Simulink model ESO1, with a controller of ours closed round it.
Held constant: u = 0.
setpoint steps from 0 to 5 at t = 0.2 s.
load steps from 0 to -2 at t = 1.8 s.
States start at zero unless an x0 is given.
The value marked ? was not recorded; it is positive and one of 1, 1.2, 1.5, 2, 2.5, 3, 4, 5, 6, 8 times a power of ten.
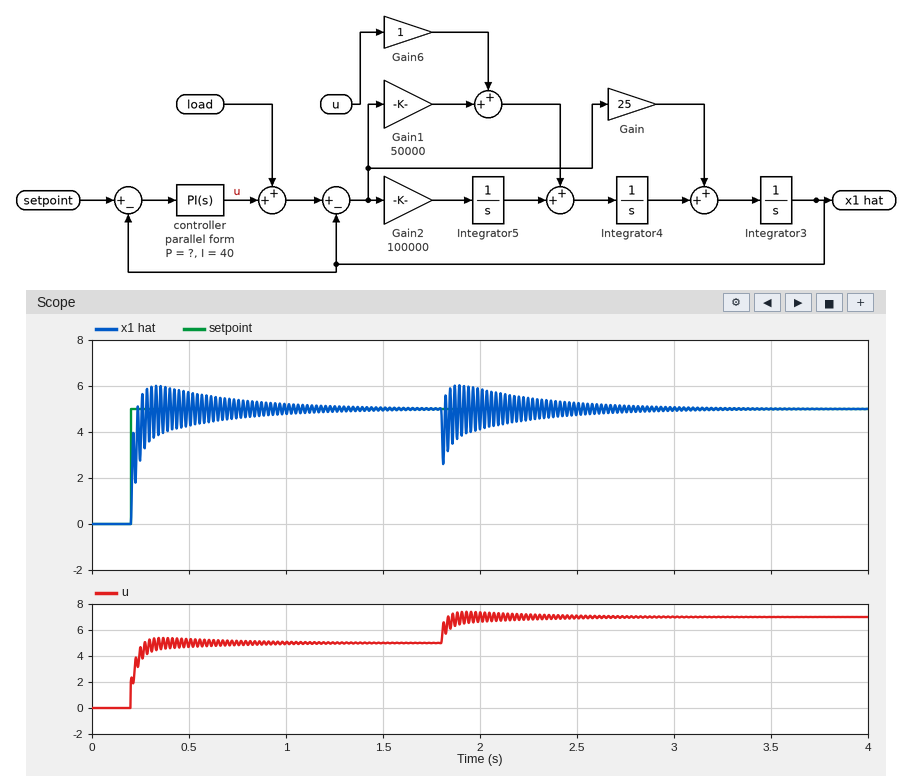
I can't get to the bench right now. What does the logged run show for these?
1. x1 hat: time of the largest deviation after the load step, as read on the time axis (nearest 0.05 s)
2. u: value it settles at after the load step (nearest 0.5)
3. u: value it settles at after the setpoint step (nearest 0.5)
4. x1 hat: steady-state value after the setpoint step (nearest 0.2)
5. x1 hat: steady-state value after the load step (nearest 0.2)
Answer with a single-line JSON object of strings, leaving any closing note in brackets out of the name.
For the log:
{"x1 hat: time of the largest deviation after the load step, as read on the time axis": "1.80 s", "u: value it settles at after the load step": "7.0", "u: value it settles at after the setpoint step": "5.0", "x1 hat: steady-state value after the setpoint step": "5.0", "x1 hat: steady-state value after the load step": "5.0"}
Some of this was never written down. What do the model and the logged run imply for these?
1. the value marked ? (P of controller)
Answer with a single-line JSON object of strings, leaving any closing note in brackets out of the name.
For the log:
{"the value marked ?": "0.4"}
